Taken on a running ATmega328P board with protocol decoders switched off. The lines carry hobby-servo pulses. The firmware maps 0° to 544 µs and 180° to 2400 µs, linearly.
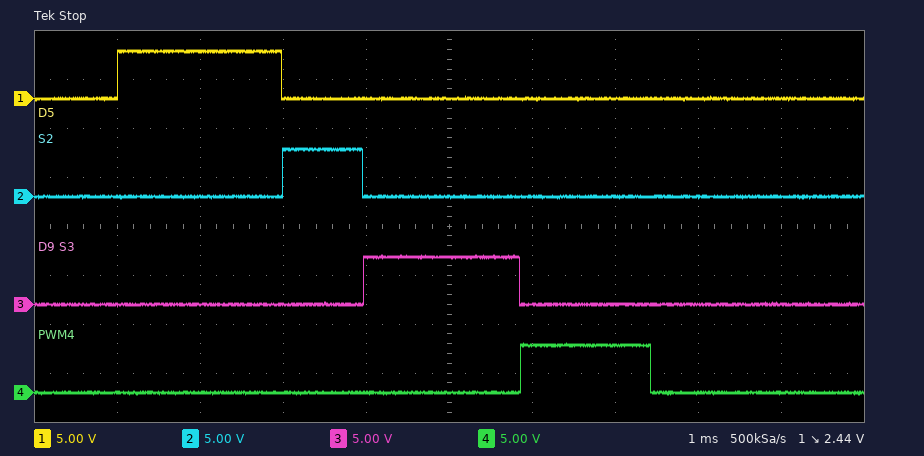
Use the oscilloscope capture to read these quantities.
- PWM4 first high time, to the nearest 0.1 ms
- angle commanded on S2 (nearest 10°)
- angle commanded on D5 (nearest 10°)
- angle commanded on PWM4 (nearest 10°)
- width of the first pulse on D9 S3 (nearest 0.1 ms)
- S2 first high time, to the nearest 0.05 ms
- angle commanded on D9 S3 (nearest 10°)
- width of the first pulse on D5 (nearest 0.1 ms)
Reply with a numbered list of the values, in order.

1. 1.6 ms
2. 40°
3. 140°
4. 100°
5. 1.9 ms
6. 0.95 ms
7. 130°
8. 2.0 ms
